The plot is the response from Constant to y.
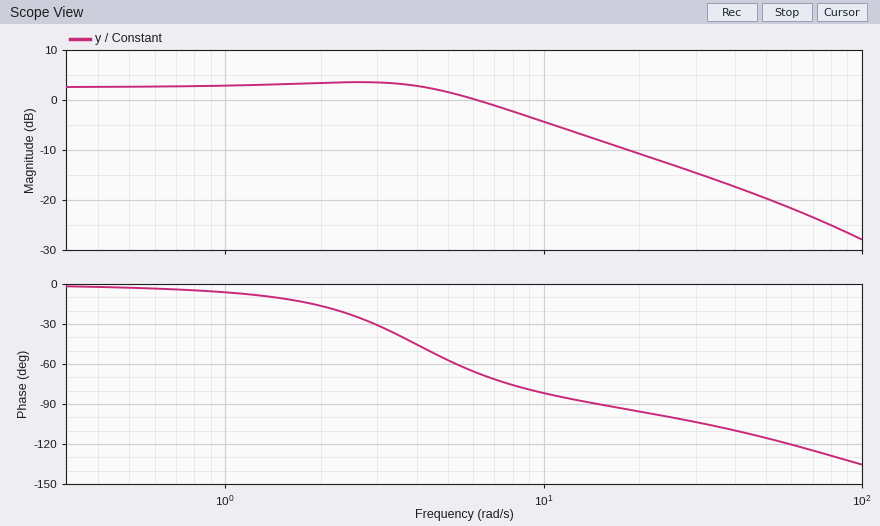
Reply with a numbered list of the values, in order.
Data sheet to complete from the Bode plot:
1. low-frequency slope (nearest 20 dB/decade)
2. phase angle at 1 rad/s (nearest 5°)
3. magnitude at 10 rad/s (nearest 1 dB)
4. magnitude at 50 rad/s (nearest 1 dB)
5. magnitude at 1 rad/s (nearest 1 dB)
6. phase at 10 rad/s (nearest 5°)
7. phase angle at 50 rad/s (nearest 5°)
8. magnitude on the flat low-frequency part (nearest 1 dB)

1. 0 dB/decade
2. -5°
3. -4 dB
4. -20 dB
5. 3 dB
6. -80°
7. -115°
8. 3 dB
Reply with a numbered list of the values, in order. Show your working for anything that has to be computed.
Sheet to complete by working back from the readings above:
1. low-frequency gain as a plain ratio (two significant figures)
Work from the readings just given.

1. 10^(3 / 20) = 1.4
